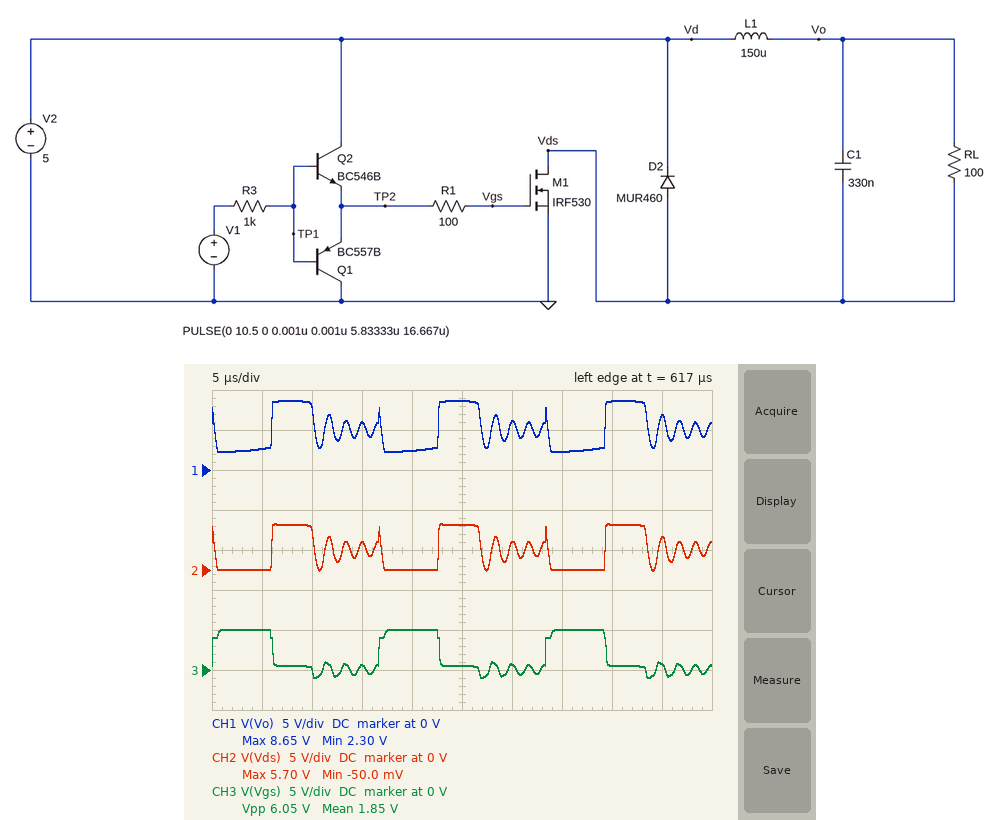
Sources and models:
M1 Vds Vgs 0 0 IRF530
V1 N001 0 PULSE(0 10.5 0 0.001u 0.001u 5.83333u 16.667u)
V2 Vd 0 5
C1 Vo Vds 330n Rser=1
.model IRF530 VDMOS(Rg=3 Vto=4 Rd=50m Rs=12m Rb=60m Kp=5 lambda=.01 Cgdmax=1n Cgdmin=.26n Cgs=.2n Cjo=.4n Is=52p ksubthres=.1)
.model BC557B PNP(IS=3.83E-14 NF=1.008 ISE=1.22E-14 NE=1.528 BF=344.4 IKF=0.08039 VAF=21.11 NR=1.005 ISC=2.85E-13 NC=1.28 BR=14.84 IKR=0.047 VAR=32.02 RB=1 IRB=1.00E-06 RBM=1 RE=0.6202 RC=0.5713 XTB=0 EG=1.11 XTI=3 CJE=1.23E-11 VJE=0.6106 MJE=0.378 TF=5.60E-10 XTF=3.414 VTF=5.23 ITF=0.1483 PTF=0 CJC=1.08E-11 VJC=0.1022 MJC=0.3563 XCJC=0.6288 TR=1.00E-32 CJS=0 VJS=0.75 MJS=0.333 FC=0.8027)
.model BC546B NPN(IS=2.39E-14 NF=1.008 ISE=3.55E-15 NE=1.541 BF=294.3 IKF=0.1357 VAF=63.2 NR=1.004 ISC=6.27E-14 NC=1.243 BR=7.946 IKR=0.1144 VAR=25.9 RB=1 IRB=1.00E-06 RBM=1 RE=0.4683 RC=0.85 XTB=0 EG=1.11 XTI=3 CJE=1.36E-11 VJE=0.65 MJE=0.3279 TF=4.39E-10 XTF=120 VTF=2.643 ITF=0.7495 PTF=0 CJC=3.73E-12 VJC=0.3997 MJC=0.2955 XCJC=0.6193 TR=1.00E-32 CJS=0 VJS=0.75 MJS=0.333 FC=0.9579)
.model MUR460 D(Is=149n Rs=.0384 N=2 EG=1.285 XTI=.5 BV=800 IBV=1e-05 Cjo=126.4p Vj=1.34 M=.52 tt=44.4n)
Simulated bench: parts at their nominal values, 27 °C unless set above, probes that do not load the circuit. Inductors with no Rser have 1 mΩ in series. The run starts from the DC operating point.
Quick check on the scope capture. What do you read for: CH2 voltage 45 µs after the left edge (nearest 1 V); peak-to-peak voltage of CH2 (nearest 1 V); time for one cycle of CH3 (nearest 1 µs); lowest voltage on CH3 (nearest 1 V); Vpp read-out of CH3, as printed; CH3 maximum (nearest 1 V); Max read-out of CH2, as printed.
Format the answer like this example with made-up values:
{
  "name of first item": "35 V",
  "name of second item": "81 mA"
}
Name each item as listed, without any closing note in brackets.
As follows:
{
  "CH2 voltage 45 µs after the left edge": "4 V",
  "peak-to-peak voltage of CH2": "6 V",
  "time for one cycle of CH3": "17 µs",
  "lowest voltage on CH3": "-1 V",
  "Vpp read-out of CH3, as printed": "6.05 V",
  "CH3 maximum": "5 V",
  "Max read-out of CH2, as printed": "5.70 V"
}
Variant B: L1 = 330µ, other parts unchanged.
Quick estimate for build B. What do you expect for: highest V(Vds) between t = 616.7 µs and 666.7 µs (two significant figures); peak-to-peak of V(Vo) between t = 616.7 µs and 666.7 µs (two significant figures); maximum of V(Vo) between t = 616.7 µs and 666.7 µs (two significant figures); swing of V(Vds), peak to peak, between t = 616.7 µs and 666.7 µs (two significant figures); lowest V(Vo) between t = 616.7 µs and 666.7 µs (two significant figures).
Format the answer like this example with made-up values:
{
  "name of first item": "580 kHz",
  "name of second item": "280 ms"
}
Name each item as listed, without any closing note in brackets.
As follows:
{
  "highest V(Vds) between t = 616.7 µs and 666.7 µs": "5.7 V",
  "peak-to-peak of V(Vo) between t = 616.7 µs and 666.7 µs": "6.0 V",
  "maximum of V(Vo) between t = 616.7 µs and 666.7 µs": "7.8 V",
  "swing of V(Vds), peak to peak, between t = 616.7 µs and 666.7 µs": "5.7 V",
  "lowest V(Vo) between t = 616.7 µs and 666.7 µs": "1.8 V"
}
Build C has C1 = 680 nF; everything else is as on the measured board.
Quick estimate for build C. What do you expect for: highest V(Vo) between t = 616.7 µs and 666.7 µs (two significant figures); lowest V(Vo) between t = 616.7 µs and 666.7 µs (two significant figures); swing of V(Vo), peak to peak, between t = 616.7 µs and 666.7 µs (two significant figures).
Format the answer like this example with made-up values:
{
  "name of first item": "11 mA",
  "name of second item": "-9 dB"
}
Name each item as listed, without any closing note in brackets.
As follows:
{
  "highest V(Vo) between t = 616.7 µs and 666.7 µs": "8.4 V",
  "lowest V(Vo) between t = 616.7 µs and 666.7 µs": "2.4 V",
  "swing of V(Vo), peak to peak, between t = 616.7 µs and 666.7 µs": "6.0 V"
}
